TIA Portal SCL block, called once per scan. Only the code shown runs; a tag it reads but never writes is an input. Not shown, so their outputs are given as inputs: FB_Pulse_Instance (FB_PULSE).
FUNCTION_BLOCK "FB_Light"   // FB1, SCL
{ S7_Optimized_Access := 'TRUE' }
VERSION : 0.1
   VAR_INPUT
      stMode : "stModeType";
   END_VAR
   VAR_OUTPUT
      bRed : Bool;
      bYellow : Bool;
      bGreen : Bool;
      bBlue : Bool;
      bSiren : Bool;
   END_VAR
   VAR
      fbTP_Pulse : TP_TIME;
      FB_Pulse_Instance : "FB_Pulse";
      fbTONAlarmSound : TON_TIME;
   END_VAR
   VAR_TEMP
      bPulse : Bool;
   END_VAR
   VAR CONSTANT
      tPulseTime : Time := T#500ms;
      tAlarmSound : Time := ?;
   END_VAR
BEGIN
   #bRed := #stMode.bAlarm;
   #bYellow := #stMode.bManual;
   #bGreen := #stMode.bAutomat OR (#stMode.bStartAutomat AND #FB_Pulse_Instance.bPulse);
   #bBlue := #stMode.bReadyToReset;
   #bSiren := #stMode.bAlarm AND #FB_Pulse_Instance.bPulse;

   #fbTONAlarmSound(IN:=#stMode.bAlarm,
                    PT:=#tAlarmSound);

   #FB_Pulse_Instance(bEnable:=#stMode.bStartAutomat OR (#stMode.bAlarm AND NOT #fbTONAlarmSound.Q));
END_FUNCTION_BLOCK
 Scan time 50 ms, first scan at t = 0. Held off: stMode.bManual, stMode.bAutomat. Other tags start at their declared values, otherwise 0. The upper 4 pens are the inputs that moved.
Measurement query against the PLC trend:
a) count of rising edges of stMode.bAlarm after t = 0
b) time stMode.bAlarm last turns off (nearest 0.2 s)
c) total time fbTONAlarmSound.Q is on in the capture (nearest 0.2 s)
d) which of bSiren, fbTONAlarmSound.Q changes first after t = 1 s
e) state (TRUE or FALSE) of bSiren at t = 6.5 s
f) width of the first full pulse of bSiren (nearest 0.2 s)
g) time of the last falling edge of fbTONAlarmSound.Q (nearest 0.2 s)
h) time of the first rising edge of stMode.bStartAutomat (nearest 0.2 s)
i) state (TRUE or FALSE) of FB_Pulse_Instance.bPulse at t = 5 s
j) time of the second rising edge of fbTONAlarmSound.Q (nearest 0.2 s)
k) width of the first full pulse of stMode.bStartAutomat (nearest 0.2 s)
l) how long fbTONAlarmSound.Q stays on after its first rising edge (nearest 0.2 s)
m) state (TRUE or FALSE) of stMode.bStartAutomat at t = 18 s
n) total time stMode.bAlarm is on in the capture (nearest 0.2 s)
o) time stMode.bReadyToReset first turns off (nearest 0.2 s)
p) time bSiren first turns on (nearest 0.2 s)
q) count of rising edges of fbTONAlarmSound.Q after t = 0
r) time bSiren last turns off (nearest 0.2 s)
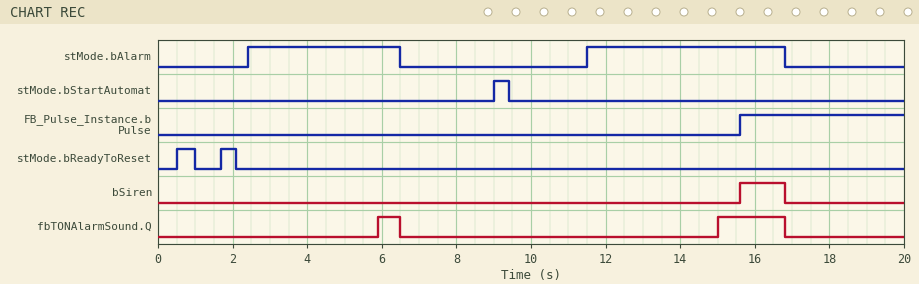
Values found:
2
16.8 s
2.4 s
fbTONAlarmSound.Q
FALSE
1.2 s
16.8 s
9.0 s
FALSE
15.0 s
0.4 s
0.6 s
FALSE
9.4 s
1.0 s
15.6 s
2
16.8 s
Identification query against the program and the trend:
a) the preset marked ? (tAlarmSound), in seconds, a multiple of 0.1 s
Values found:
3.5 s
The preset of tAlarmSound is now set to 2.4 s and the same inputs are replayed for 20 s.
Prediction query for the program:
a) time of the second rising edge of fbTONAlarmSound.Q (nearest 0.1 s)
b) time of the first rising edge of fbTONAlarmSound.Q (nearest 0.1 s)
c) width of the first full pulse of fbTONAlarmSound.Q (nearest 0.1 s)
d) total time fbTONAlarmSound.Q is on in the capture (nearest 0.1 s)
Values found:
13.9 s
4.8 s
1.7 s
4.6 s
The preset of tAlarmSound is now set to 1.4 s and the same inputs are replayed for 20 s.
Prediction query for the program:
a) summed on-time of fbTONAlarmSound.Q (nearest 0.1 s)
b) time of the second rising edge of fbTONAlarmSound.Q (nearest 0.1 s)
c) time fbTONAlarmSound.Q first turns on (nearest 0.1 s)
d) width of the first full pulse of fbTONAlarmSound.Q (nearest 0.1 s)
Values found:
6.6 s
12.9 s
3.8 s
2.7 s
